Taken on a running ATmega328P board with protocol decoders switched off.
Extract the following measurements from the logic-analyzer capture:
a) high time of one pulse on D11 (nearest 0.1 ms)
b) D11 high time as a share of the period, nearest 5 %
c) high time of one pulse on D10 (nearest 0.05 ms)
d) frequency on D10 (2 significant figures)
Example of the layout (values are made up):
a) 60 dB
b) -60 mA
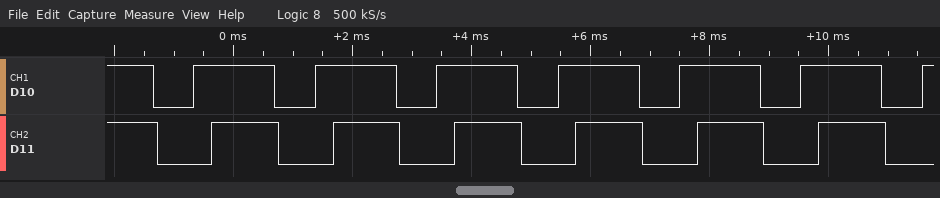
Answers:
a) 1.1 ms
b) 55 %
c) 1.35 ms
d) 490 Hz
